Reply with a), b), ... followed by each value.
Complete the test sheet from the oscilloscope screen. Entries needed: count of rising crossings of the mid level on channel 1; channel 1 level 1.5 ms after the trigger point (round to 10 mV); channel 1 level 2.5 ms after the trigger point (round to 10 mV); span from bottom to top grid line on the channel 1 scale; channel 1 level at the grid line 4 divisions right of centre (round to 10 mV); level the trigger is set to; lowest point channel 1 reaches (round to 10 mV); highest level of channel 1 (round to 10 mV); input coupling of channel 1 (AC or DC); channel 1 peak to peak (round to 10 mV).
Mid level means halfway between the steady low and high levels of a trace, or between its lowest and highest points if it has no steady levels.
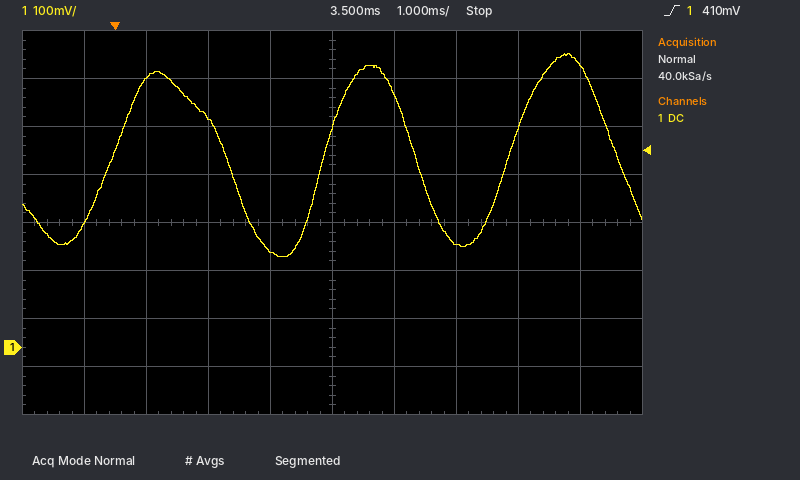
a) 3
b) 480 mV
c) 200 mV
d) 800 mV
e) 590 mV
f) 410 mV
g) 190 mV
h) 610 mV
i) DC
j) 420 mV
